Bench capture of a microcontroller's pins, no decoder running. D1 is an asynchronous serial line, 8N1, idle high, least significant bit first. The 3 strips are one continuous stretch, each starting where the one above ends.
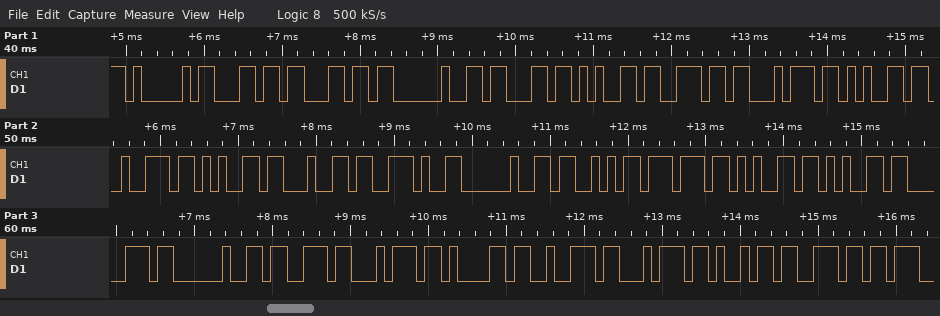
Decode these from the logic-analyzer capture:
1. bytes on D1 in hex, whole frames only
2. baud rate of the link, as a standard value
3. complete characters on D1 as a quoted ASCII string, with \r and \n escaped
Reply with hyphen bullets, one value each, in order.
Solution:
- 41 6C 6C 20 63 65 6E 74 65 72 65 64 2E 20 53 77 65 65 70 20 73 74 61 72 74 69 6E
- 9600 baud
- "All centered. Sweep startin"
